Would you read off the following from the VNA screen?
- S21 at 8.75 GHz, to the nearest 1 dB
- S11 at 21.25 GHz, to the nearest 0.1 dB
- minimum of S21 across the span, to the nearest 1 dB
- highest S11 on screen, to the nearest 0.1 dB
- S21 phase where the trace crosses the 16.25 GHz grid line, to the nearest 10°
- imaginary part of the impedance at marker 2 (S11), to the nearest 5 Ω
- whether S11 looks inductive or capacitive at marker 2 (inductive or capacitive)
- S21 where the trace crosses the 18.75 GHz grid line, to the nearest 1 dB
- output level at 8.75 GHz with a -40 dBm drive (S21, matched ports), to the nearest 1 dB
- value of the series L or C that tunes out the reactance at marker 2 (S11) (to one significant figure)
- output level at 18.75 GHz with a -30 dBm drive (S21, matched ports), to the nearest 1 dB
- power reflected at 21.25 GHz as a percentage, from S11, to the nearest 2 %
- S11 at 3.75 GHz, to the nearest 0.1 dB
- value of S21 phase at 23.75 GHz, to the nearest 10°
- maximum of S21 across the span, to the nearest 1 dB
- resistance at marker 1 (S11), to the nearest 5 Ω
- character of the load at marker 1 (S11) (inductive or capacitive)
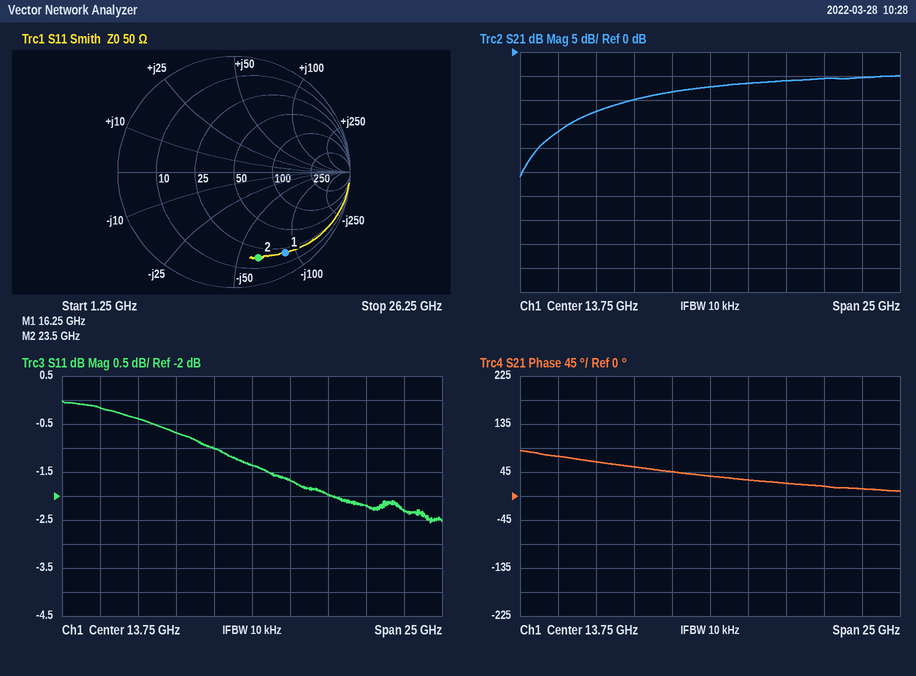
-10 dB
-2.2 dB
-26 dB
0.0 dB
30°
-65 Ω
capacitive
-6 dB
-50 dBm
400 pH
-36 dBm
60 %
-0.2 dB
10°
-5 dB
20 Ω
capacitive
